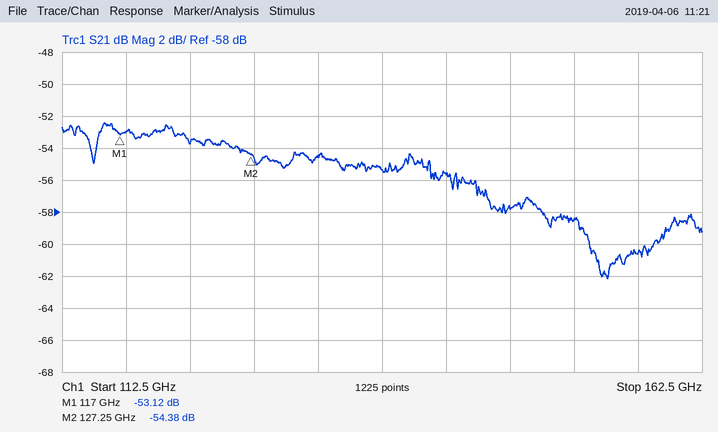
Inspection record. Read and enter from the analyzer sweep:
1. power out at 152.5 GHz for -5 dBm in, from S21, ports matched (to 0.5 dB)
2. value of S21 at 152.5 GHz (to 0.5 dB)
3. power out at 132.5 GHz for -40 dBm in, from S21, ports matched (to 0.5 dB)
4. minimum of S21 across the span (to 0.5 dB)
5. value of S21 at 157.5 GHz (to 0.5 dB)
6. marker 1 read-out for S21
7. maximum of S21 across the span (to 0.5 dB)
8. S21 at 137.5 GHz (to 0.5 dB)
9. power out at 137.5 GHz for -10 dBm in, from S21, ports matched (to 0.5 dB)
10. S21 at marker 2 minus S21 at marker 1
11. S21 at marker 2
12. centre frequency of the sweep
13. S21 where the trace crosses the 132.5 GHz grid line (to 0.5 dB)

-63.5 dBm
-58.5 dB
-94.5 dBm
-62.0 dB
-60.5 dB
-53.12 dB
-52.5 dB
-55.5 dB
-65.5 dBm
-1.26 dB
-54.38 dB
137.5 GHz
-54.5 dB
